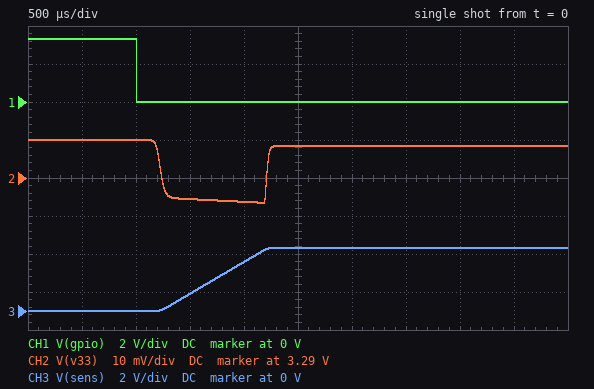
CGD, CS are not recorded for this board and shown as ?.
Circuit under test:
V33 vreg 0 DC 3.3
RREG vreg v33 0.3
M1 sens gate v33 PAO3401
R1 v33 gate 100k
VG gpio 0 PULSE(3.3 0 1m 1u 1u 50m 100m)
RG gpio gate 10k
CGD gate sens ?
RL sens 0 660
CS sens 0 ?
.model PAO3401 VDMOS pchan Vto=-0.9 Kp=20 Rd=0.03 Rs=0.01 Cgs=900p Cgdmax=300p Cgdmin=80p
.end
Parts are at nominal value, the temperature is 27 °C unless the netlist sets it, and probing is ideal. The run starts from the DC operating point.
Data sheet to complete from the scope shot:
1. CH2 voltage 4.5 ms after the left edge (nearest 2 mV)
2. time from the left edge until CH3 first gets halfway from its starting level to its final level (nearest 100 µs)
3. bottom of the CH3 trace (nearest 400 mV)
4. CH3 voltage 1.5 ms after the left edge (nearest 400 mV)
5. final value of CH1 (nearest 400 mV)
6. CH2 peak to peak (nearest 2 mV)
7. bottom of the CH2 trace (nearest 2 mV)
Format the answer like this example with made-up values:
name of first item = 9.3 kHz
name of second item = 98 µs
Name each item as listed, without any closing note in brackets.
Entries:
CH2 voltage 4.5 ms after the left edge = 3.298 V
time from the left edge until CH3 first gets halfway from its starting level to its final level = 1.7 ms
bottom of the CH3 trace = 0 V
CH3 voltage 1.5 ms after the left edge = 800 mV
final value of CH1 = 0 V
CH2 peak to peak = 16 mV
bottom of the CH2 trace = 3.284 V
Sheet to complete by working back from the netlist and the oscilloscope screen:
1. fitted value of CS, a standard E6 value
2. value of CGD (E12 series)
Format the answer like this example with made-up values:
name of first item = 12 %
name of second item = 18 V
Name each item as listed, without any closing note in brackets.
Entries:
fitted value of CS, a standard E6 value = 15 µF
value of CGD = 68 nF
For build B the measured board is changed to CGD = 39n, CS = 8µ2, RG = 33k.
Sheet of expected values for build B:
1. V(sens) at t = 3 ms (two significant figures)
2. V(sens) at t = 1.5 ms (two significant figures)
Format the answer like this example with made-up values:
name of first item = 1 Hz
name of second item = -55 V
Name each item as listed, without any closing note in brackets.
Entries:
V(sens) at t = 3 ms = 2.7 V
V(sens) at t = 1.5 ms = 170 mV
